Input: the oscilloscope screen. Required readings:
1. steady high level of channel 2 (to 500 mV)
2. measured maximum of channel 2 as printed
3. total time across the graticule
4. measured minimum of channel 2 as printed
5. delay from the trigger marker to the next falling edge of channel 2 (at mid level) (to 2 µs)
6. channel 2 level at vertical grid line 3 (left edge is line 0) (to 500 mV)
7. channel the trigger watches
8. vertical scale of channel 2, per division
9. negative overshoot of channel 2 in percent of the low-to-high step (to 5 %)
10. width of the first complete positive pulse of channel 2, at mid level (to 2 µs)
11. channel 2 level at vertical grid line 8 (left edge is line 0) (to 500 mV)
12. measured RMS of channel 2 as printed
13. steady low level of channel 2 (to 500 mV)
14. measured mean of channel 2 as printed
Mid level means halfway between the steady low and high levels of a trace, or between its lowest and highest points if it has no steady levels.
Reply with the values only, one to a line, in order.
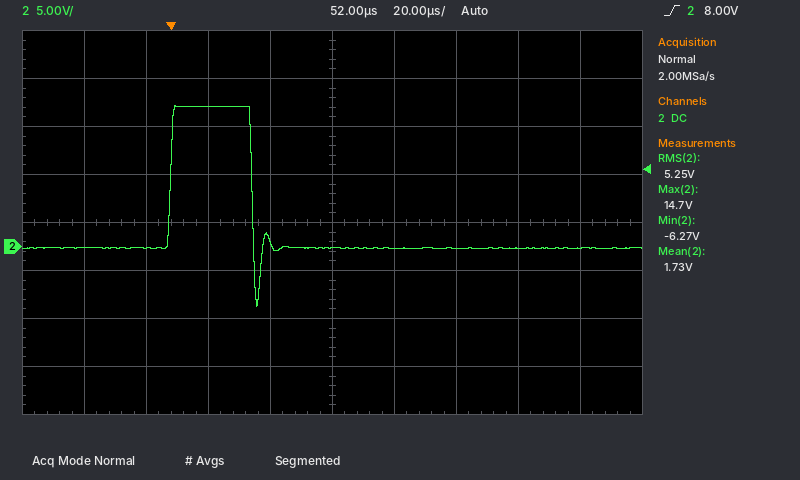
14.5 V
14.7 V
200 µs
-6.27 V
26 µs
14.5 V
channel 2
5 V
40 %
26 µs
0.0 V
5.25 V
0.0 V
1.73 V
